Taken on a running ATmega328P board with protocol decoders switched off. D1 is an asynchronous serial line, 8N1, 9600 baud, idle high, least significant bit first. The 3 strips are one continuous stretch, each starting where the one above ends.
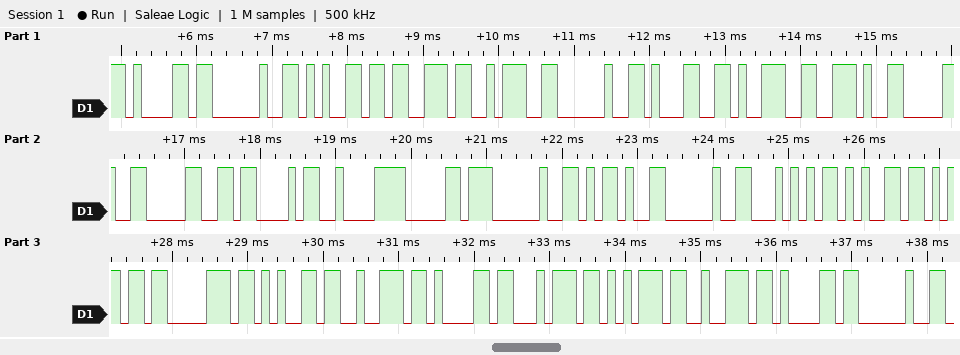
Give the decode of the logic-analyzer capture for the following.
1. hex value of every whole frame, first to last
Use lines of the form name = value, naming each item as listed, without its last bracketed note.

hex value of every whole frame, first to last = 61 20 65 73 3A 20 31 39 2E 30 30 43 C2 B0 20 2D 20 54 65 6D 70 65 72 61 74 75 72 61 20
